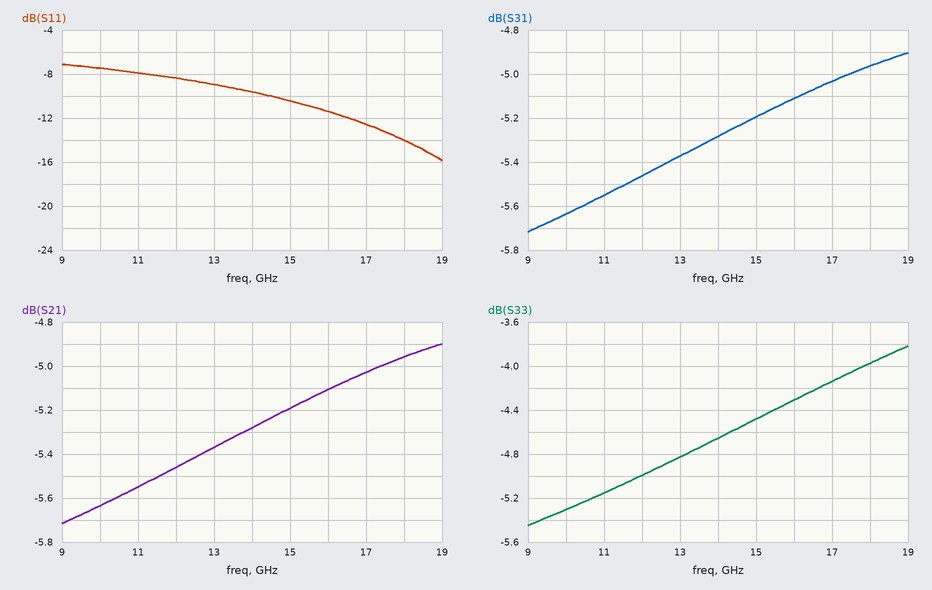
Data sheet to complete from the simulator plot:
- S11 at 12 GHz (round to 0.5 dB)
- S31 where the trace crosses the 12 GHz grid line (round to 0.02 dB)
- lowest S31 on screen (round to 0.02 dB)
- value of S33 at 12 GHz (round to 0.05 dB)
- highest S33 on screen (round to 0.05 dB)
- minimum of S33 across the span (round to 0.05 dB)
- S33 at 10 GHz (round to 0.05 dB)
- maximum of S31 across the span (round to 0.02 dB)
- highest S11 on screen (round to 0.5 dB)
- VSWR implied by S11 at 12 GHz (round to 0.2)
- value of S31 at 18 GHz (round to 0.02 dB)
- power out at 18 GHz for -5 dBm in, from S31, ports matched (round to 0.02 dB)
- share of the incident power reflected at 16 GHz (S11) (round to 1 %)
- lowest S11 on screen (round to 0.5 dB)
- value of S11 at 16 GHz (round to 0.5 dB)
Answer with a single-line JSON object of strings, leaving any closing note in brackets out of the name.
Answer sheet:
{"S11 at 12 GHz": "-8.5 dB", "S31 where the trace crosses the 12 GHz grid line": "-5.46 dB", "lowest S31 on screen": "-5.72 dB", "value of S33 at 12 GHz": "-5.00 dB", "highest S33 on screen": "-3.80 dB", "minimum of S33 across the span": "-5.45 dB", "S33 at 10 GHz": "-5.30 dB", "maximum of S31 across the span": "-4.90 dB", "highest S11 on screen": "-7.0 dB", "VSWR implied by S11 at 12 GHz": "2.2", "value of S31 at 18 GHz": "-4.96 dB", "power out at 18 GHz for -5 dBm in, from S31, ports matched": "-9.96 dBm", "share of the incident power reflected at 16 GHz (S11)": "7 %", "lowest S11 on screen": "-16.0 dB", "value of S11 at 16 GHz": "-11.5 dB"}
